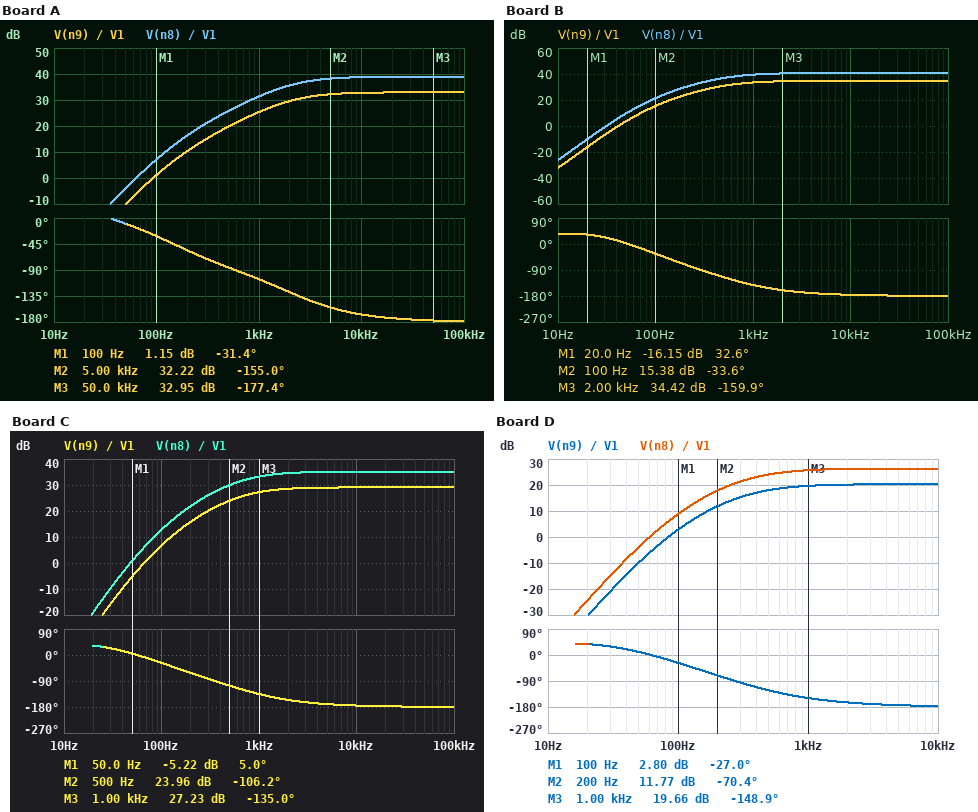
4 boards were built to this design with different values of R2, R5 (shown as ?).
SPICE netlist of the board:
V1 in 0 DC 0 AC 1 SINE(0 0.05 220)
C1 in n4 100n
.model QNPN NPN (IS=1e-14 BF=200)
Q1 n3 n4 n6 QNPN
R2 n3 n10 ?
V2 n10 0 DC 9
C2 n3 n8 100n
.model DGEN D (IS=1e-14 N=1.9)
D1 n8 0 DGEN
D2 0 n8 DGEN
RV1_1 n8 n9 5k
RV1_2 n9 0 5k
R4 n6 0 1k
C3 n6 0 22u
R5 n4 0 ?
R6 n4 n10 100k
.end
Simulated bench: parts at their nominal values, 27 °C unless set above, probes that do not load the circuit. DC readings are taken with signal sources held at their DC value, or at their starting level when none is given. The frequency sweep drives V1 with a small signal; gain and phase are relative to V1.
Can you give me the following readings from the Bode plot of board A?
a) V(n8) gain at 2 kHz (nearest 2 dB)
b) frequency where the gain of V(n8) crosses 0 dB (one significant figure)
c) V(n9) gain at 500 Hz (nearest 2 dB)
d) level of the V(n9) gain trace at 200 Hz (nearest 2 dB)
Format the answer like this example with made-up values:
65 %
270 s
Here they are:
36 dB
60 Hz
20 dB
10 dB
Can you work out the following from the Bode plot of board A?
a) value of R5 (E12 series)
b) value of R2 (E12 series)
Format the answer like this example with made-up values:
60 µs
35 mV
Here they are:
150 kΩ
680 Ω
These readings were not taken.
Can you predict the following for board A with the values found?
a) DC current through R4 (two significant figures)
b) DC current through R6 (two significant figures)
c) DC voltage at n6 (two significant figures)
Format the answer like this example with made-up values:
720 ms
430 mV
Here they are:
3.6 mA
47 µA
3.6 V
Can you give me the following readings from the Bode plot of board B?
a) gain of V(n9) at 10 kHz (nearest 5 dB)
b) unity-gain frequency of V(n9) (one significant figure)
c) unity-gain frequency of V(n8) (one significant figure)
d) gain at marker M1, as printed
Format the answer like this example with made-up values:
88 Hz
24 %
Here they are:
35 dB
40 Hz
30 Hz
-16.15 dB
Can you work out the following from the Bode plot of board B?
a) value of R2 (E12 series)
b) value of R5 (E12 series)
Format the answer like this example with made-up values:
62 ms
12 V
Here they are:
4.7 kΩ
22 kΩ
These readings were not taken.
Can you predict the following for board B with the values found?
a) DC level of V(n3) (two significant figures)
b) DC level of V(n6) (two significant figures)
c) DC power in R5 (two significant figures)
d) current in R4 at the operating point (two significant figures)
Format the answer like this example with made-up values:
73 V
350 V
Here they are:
4.8 V
890 mV
110 µW
890 µA
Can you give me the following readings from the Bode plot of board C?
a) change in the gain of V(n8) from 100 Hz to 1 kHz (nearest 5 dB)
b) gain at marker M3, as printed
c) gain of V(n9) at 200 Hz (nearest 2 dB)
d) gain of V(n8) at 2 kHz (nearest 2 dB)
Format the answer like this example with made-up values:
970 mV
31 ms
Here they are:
20 dB
27.23 dB
16 dB
34 dB
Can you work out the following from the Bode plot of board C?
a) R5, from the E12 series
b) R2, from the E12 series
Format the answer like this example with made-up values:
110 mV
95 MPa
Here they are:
27 kΩ
1.5 kΩ
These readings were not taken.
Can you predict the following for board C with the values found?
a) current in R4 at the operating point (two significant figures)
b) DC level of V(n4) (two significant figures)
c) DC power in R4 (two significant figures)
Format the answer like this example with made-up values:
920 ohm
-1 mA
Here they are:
1.1 mA
1.8 V
1.3 mW
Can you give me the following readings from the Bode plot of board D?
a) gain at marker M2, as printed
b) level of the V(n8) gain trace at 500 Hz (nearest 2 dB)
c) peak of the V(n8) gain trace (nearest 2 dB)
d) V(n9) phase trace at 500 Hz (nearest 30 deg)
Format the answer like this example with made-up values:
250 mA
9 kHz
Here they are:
11.77 dB
24 dB
26 dB
-120 deg
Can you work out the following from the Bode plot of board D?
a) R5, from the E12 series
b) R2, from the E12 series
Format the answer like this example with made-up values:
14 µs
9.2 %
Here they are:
15 kΩ
1.2 kΩ
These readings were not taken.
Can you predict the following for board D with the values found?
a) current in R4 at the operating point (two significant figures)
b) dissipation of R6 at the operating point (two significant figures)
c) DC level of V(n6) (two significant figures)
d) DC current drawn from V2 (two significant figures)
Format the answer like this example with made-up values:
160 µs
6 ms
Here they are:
500 µA
620 µW
500 mV
580 µA
